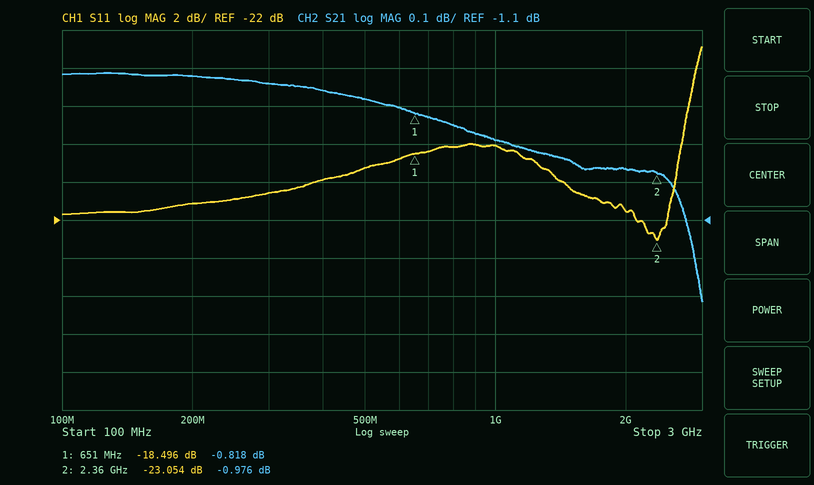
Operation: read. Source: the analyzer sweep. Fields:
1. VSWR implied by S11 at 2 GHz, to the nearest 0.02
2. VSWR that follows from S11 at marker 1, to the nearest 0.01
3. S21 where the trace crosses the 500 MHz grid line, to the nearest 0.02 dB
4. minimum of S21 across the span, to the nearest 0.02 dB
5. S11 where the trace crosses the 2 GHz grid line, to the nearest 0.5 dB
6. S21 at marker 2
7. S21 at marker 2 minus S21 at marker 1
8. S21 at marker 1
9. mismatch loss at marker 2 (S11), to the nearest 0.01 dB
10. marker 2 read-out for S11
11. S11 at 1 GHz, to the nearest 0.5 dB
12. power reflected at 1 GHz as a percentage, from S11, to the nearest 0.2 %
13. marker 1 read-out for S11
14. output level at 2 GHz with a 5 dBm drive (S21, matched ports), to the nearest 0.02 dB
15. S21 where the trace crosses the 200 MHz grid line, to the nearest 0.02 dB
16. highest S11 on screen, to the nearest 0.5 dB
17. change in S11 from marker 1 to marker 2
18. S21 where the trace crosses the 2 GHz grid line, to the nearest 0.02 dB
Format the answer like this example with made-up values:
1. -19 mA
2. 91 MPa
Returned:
1. 1.18
2. 1.27
3. -0.78 dB
4. -1.32 dB
5. -21.5 dB
6. -0.976 dB
7. -0.158 dB
8. -0.818 dB
9. 0.02 dB
10. -23.054 dB
11. -18.0 dB
12. 1.6 %
13. -18.496 dB
14. 4.04 dBm
15. -0.72 dB
16. -13.0 dB
17. -4.558 dB
18. -0.96 dB
